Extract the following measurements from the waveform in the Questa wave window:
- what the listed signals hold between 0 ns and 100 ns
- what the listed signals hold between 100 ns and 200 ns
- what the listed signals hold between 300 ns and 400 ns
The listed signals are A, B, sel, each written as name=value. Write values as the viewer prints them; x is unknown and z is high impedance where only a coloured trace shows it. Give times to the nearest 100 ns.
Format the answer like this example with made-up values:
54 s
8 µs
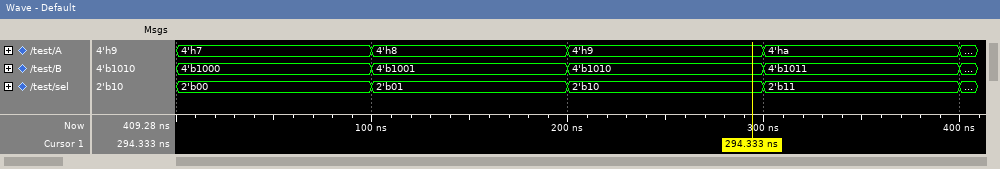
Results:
A=4'h7, B=4'b1000, sel=2'b00
A=4'h8, B=4'b1001, sel=2'b01
A=4'ha, B=4'b1011, sel=2'b11
